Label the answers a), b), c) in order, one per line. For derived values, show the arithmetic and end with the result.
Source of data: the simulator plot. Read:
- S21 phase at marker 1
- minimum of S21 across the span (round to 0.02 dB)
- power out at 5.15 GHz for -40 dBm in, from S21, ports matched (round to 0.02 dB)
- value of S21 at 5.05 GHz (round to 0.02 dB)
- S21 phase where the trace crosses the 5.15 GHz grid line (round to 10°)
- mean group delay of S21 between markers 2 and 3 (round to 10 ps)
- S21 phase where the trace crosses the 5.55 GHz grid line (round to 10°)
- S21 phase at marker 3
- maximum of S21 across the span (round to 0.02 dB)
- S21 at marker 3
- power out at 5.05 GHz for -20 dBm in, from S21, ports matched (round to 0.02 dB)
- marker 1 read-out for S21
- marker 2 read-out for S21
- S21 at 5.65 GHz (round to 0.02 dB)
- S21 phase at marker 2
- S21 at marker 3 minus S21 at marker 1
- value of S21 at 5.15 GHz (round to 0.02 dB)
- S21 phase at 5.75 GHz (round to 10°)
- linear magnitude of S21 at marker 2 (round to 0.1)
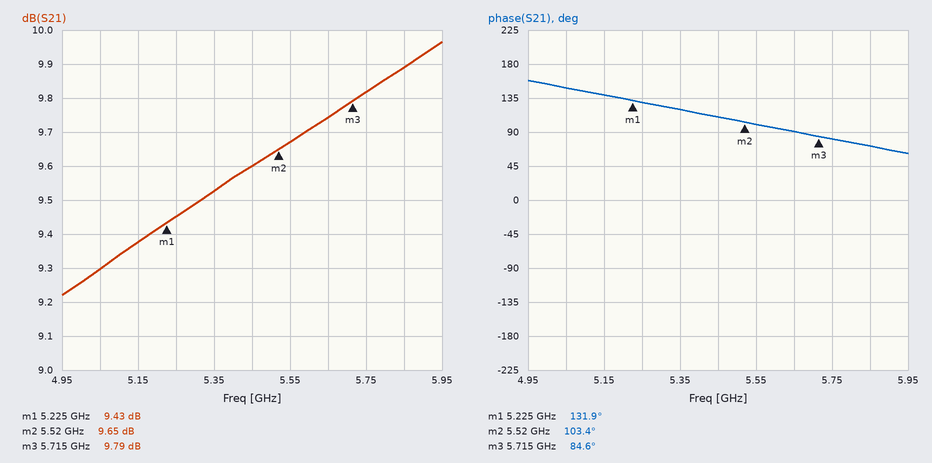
a) 131.9°
b) 9.22 dB
c) -40 dBm + (9.38 dB) = -30.62 dBm
d) 9.30 dB
e) 140°
f) −(84.6° − (103.4°))/(360° × 195 MHz) ≈ 268 ps, so 270 ps to the nearest 10 ps
g) 100°
h) 84.6°
i) 9.96 dB
j) 9.79 dB
k) -20 dBm + (9.30 dB) = -10.70 dBm
l) 9.43 dB
m) 9.65 dB
n) 9.74 dB
o) 103.4°
p) 9.79 − (9.43) = 0.36 dB
q) 9.38 dB
r) 80°
s) 10^(9.65/20) ≈ 3.0
